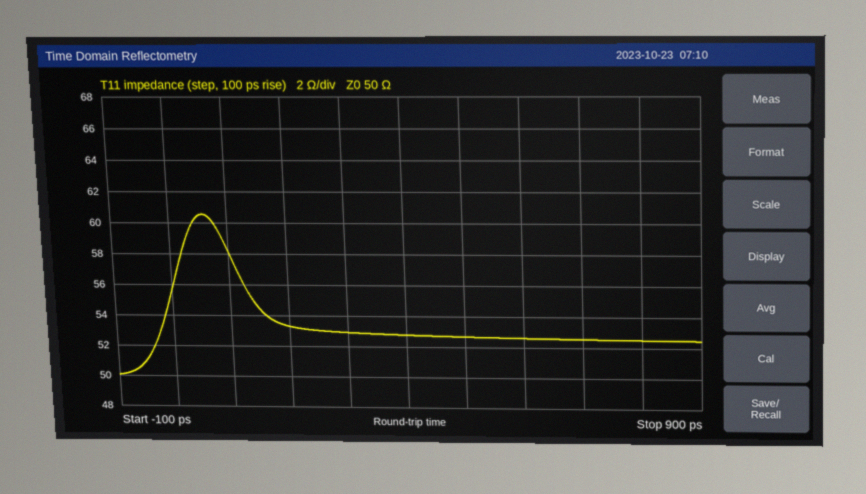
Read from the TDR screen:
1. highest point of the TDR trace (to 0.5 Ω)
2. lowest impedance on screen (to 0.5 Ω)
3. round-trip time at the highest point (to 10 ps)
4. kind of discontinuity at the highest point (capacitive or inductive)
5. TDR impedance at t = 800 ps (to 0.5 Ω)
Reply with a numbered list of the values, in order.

1. 60.5 Ω
2. 50.0 Ω
3. 60 ps
4. inductive
5. 52.5 Ω
